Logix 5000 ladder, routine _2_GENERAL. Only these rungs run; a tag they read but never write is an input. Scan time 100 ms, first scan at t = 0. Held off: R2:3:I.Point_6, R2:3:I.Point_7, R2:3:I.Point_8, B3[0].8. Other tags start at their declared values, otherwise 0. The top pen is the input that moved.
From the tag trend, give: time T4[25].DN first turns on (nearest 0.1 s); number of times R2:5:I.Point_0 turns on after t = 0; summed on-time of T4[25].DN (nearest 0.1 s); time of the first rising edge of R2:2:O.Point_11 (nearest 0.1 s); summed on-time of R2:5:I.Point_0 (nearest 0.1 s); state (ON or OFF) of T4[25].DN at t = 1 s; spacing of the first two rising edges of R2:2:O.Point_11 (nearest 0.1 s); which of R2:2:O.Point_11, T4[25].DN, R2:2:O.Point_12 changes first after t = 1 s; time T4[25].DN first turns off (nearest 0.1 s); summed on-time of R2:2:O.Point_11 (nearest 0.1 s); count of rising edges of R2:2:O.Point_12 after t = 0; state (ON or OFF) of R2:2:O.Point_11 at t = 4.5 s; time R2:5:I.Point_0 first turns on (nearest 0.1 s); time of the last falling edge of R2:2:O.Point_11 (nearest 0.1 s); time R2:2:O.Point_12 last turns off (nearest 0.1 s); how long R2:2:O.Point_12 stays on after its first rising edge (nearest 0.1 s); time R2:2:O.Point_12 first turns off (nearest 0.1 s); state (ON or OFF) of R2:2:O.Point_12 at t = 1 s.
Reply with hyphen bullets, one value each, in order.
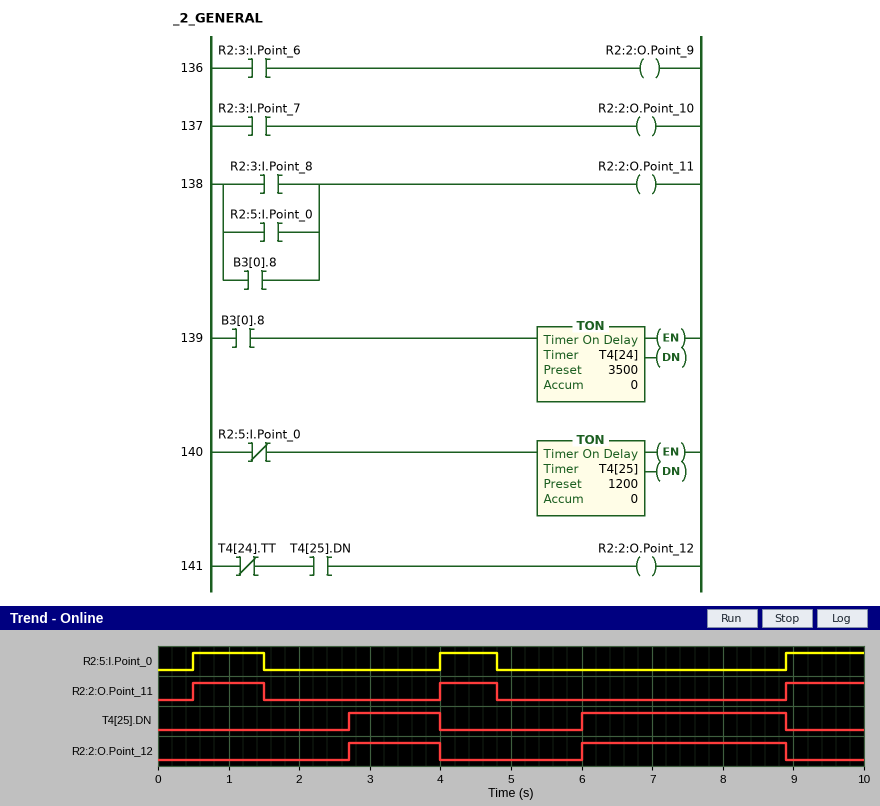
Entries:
- 2.7 s
- 3
- 4.2 s
- 0.5 s
- 2.9 s
- OFF
- 3.5 s
- R2:2:O.Point_11
- 4.0 s
- 2.9 s
- 2
- ON
- 0.5 s
- 4.8 s
- 8.9 s
- 1.3 s
- 4.0 s
- OFF
